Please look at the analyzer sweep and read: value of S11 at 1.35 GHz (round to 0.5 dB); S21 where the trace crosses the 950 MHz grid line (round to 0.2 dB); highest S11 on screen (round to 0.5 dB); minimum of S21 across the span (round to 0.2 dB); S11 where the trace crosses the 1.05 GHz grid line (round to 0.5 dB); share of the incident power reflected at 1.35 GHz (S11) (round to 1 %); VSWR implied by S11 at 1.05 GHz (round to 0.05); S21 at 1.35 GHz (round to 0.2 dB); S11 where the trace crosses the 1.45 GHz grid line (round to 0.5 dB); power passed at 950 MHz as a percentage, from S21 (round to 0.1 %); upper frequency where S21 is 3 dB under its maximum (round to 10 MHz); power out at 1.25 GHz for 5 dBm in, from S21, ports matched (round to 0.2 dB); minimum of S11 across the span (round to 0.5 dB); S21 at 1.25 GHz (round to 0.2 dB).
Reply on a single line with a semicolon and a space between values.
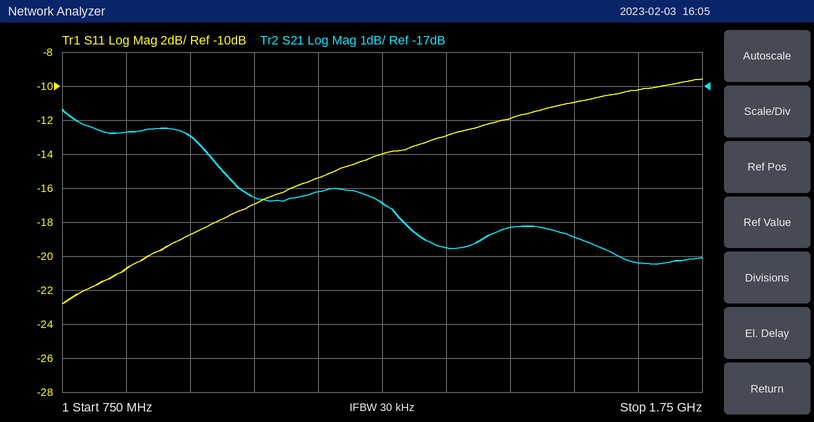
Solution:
-13.0 dB; -18.4 dB; -9.5 dB; -22.2 dB; -17.0 dB; 5 %; 1.35; -21.8 dB; -12.0 dB; 1.4 %; 1.27 GHz; -15.4 dBm; -23.0 dB; -20.4 dB
